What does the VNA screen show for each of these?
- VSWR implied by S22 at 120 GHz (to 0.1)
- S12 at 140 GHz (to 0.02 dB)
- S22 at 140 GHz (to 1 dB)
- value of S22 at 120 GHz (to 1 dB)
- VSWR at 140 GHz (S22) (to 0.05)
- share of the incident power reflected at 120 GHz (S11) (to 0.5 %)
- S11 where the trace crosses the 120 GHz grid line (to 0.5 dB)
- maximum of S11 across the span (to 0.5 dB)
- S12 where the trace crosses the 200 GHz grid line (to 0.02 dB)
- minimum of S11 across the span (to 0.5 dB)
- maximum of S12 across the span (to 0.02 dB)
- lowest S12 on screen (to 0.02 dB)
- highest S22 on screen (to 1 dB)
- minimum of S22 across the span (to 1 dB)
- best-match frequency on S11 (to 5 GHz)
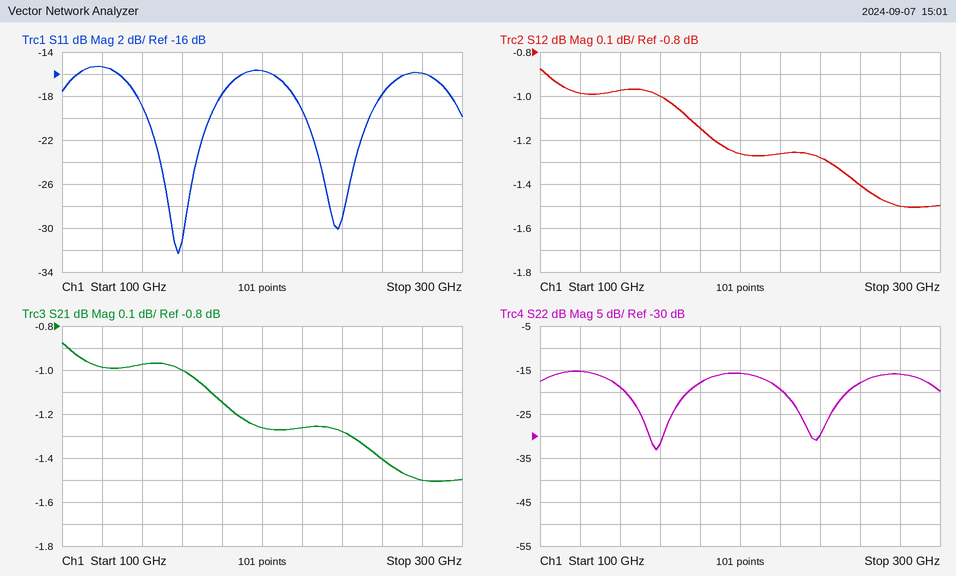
1.4
-0.98 dB
-19 dB
-15 dB
1.25
3.0 %
-15.5 dB
-15.5 dB
-1.26 dB
-32.5 dB
-0.88 dB
-1.50 dB
-15 dB
-33 dB
160 GHz
